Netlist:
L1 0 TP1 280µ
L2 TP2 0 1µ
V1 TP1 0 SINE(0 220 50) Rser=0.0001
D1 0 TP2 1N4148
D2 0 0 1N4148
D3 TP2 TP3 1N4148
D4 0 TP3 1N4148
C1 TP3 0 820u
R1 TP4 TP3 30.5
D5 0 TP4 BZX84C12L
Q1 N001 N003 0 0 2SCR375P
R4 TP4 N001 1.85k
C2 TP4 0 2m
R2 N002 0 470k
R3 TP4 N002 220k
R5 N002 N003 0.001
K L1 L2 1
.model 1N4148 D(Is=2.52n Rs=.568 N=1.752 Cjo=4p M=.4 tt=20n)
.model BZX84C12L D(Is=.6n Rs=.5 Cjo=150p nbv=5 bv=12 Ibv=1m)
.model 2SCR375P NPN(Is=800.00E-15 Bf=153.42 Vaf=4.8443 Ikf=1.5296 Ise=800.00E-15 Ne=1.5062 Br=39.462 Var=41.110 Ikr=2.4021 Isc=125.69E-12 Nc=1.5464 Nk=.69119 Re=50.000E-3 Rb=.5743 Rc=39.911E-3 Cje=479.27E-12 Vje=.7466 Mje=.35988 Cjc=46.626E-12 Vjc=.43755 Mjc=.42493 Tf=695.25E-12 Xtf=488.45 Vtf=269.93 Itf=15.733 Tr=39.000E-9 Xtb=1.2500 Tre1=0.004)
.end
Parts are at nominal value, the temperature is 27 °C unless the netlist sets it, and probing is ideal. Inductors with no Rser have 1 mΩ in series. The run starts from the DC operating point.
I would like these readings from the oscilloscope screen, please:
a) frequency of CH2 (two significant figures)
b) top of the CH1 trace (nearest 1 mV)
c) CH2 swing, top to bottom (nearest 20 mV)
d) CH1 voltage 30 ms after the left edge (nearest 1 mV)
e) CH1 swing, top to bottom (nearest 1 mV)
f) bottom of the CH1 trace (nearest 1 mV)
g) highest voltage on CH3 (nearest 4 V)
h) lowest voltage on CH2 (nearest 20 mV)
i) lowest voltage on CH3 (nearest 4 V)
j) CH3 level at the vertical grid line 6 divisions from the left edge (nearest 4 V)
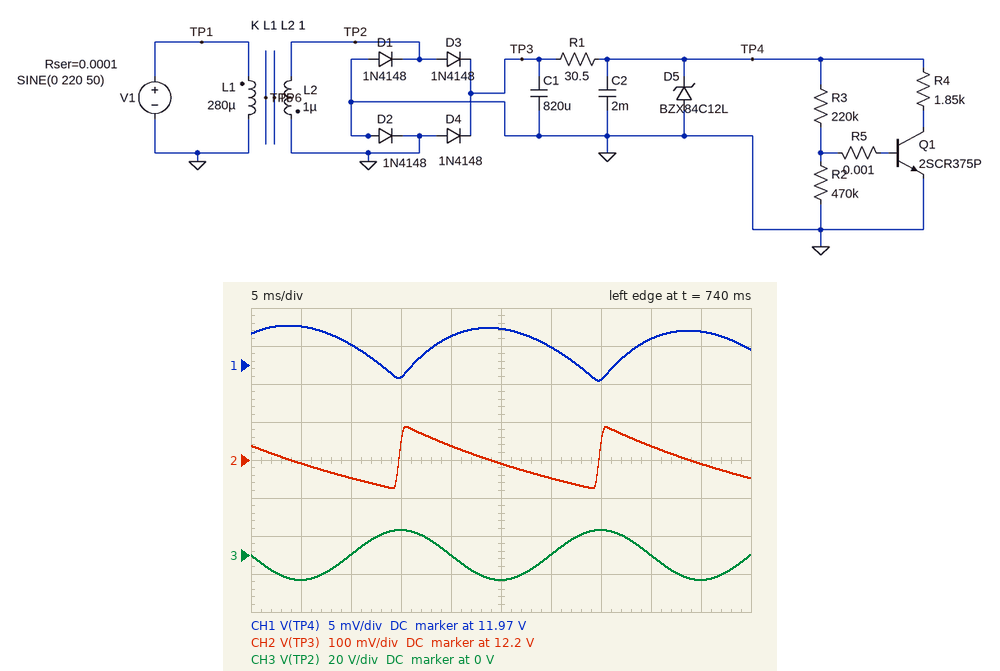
50 Hz
11.980 V
160 mV
11.977 V
7 mV
11.973 V
12 V
12.12 V
-12 V
0 V
